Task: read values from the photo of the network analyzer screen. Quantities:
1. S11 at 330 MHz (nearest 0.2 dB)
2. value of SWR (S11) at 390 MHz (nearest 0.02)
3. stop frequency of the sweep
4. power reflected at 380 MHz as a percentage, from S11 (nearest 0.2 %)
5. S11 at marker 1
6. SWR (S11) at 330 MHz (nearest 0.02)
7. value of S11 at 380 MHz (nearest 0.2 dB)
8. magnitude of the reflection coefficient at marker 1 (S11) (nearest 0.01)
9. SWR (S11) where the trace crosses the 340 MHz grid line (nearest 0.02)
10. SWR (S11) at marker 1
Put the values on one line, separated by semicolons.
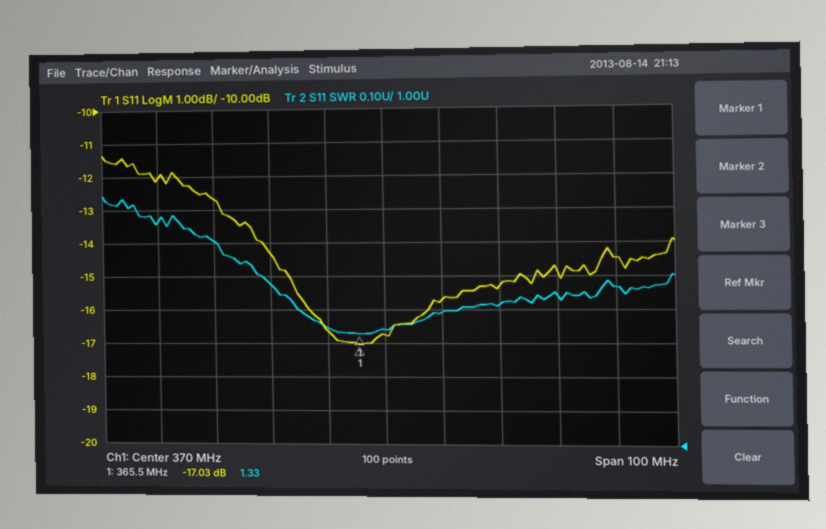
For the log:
-12.0 dB; 1.42; 420 MHz; 2.6 %; -17.03 dB; 1.66; -15.8 dB; 0.14; 1.60; 1.33
